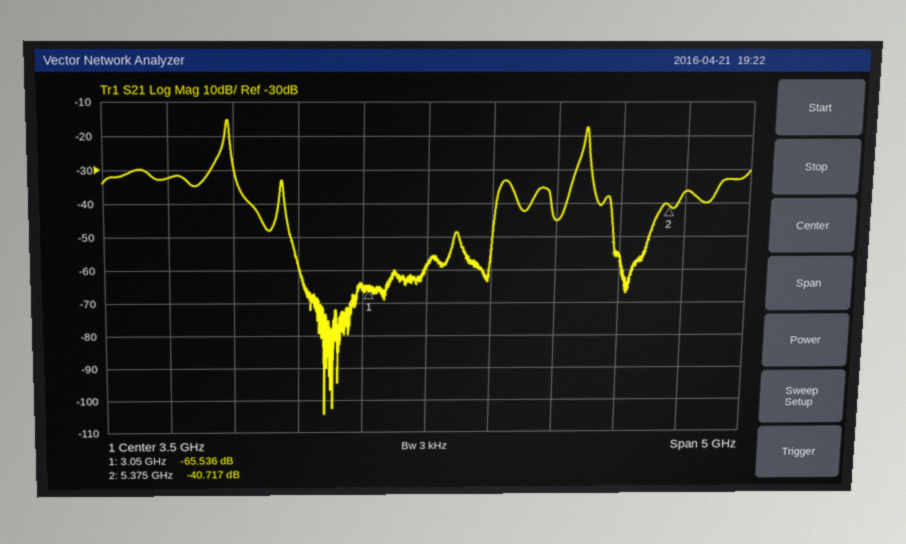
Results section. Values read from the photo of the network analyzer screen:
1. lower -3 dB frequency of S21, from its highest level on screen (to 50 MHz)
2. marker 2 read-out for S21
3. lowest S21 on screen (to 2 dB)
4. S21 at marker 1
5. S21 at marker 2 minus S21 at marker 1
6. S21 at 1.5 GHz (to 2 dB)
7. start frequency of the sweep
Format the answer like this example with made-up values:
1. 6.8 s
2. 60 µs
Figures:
1. 1.95 GHz
2. -40.717 dB
3. -104 dB
4. -65.536 dB
5. 24.819 dB
6. -32 dB
7. 1 GHz
